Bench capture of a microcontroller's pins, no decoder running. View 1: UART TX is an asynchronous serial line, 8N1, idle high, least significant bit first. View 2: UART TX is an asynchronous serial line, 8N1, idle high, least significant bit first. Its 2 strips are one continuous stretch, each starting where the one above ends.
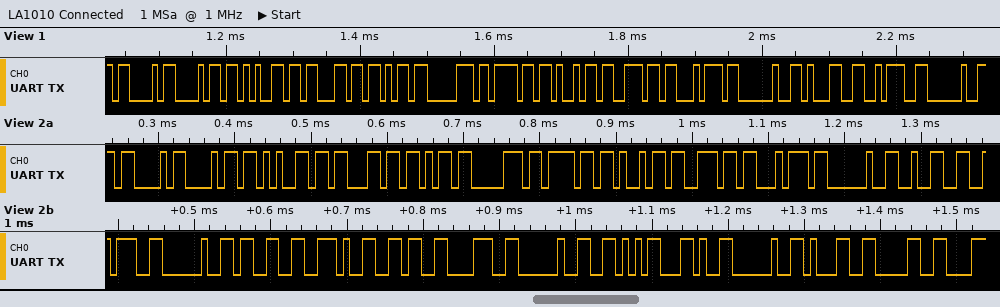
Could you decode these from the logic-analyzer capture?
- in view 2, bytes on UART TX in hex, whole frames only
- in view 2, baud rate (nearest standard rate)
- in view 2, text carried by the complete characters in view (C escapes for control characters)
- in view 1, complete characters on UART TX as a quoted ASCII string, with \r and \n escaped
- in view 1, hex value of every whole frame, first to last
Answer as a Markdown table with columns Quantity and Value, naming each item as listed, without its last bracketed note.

| Quantity | Value |
|---|---|
| in view 2, bytes on UART TX in hex, whole frames only | 43 68 65 63 6B 70 6F 69 6E 74 20 32 3A 20 33 2E 36 38 20 56 2C 20 31 30 |
| in view 2, baud rate | 115200 baud |
| in view 2, text carried by the complete characters in view | "Checkpoint 2: 3.68 V, 10" |
| in view 1, complete characters on UART TX as a quoted ASCII string, with \r and \n escaped | "Checkpoint 1: " |
| in view 1, hex value of every whole frame, first to last | 43 68 65 63 6B 70 6F 69 6E 74 20 31 3A 20 |
